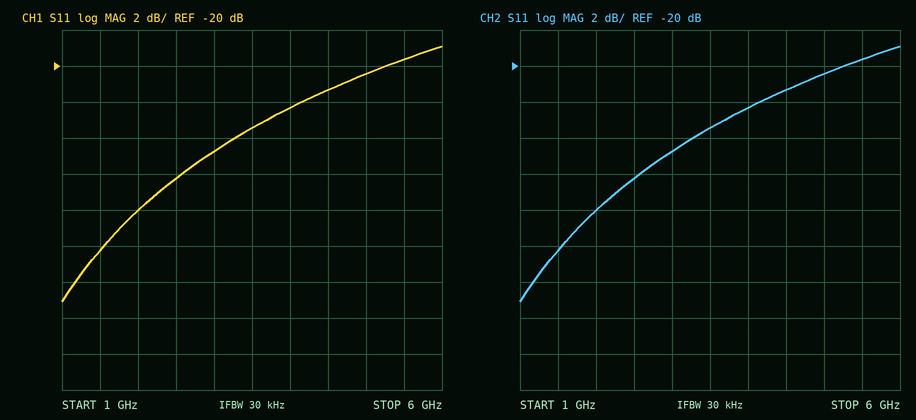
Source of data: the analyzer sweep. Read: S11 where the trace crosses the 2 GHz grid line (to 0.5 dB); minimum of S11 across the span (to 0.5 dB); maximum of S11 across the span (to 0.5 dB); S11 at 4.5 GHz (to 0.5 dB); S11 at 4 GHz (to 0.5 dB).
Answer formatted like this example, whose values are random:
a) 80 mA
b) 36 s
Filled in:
a) -28.0 dB
b) -33.0 dB
c) -19.0 dB
d) -21.5 dB
e) -22.5 dB
